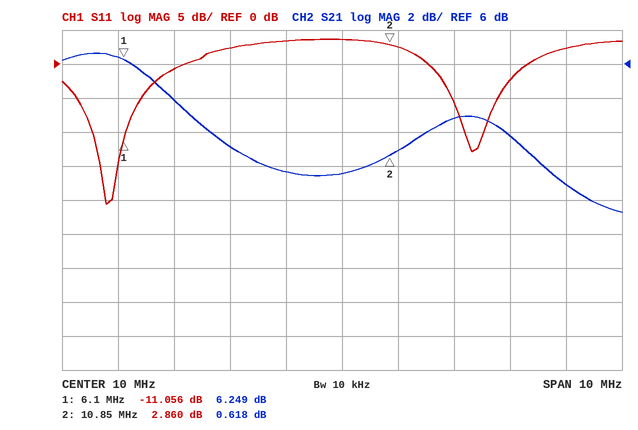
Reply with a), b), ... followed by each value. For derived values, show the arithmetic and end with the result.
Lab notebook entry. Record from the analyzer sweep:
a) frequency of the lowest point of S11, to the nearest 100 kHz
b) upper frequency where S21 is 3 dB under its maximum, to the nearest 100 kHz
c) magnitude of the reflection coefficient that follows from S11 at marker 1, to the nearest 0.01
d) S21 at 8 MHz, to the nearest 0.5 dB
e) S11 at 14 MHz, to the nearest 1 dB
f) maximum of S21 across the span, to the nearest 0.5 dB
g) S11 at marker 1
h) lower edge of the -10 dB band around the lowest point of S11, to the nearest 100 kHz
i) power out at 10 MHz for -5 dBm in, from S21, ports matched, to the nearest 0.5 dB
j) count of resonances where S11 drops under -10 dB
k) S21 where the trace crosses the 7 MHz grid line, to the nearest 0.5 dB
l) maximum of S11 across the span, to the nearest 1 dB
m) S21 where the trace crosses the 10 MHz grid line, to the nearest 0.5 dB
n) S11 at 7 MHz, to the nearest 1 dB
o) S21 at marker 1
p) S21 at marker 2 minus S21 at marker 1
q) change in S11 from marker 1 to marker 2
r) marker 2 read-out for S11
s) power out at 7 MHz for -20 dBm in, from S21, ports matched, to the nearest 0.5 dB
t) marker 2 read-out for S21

a) 5.8 MHz
b) 7.1 MHz
c) 10^(-11.056/20) ≈ 0.28
d) 1.0 dB
e) 2 dB
f) 6.5 dB
g) -11.056 dB
h) 5.5 MHz
i) -5 dBm + (-0.5 dB) = -5.5 dBm
j) 2
k) 4.0 dB
l) 4 dB
m) -0.5 dB
n) -1 dB
o) 6.249 dB
p) 0.618 − (6.249) = -5.631 dB
q) 2.86 − (-11.056) = 13.916 dB
r) 2.860 dB
s) -20 dBm + (4.0 dB) = -16.0 dBm
t) 0.618 dB
